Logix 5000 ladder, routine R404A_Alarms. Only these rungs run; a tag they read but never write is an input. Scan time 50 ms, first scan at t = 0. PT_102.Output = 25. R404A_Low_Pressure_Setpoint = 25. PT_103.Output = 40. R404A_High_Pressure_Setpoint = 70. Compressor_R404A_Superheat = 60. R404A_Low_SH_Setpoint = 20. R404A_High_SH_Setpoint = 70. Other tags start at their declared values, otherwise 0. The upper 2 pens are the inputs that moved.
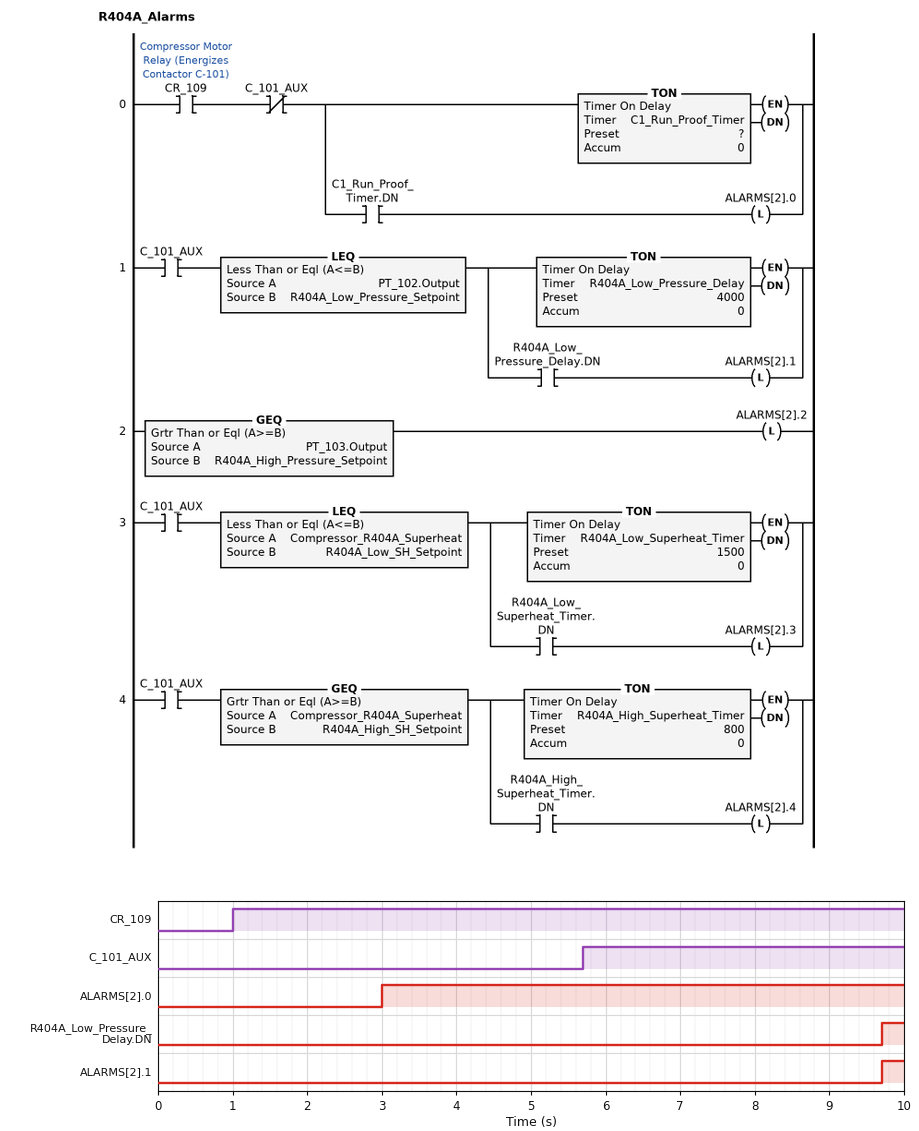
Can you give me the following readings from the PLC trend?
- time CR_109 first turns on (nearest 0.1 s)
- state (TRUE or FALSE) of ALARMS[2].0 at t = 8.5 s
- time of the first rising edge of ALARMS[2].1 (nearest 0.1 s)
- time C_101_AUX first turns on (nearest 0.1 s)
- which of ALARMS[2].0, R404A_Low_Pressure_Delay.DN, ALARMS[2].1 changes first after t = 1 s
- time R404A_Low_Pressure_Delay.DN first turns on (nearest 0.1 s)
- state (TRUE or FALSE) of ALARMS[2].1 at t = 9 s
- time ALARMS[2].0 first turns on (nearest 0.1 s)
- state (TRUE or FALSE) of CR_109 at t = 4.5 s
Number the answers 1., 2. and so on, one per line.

1. 1.0 s
2. TRUE
3. 9.7 s
4. 5.7 s
5. ALARMS[2].0
6. 9.7 s
7. FALSE
8. 3.0 s
9. TRUE
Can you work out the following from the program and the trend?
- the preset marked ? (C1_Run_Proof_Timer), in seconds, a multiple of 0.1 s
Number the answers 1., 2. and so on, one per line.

1. 2.0 s
